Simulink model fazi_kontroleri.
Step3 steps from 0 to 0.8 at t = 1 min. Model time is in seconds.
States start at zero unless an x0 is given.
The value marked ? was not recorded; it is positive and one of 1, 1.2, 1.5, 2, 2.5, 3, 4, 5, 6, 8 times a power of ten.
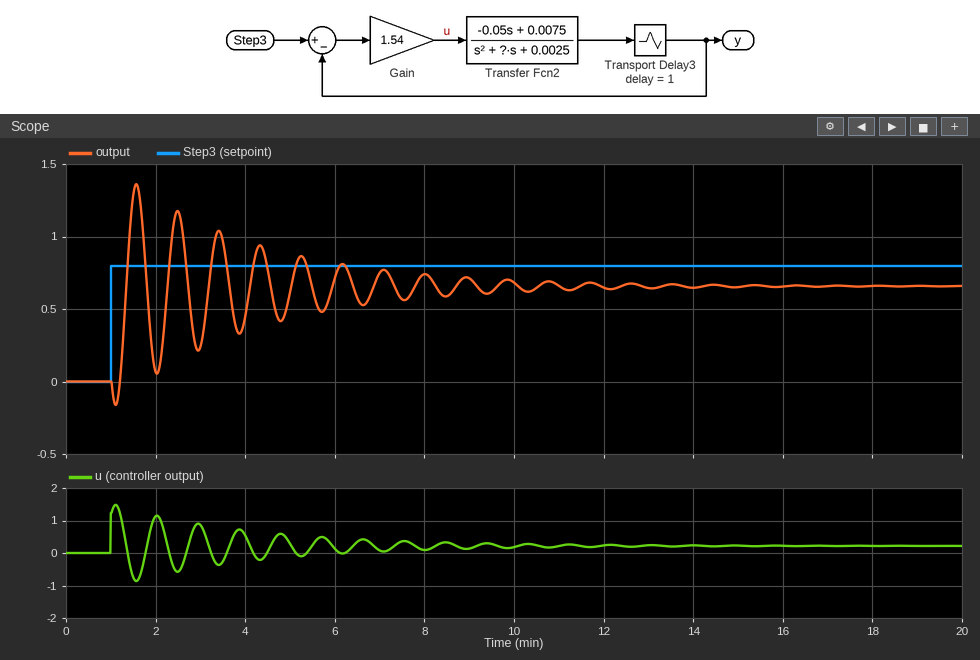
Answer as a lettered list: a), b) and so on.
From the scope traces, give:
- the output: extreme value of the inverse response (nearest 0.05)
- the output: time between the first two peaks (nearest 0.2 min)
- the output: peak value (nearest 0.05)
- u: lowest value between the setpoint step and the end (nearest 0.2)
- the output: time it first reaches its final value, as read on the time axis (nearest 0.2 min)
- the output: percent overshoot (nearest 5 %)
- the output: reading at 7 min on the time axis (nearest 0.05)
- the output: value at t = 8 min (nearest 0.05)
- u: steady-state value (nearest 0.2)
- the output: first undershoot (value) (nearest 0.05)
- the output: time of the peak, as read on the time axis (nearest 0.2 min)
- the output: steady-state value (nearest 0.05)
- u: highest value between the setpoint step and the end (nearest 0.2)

a) -0.15
b) 1.0 min
c) 1.35
d) -0.8
e) 1.4 min
f) 105 %
g) 0.75
h) 0.75
i) 0.2
j) 0.05
k) 1.6 min
l) 0.65
m) 1.4
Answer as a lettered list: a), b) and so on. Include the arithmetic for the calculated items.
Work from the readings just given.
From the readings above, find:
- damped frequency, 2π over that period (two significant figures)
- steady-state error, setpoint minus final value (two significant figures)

a) 2π / 1 = 6.3 rad/min
b) 0.8 - 0.65 = 0.15
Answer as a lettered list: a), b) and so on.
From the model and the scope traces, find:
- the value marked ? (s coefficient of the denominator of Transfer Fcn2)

a) 0.1
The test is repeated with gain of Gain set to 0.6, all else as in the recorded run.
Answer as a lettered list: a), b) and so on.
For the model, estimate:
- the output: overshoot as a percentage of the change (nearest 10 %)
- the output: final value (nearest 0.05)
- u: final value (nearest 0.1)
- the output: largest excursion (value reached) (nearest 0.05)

a) 30 %
b) 0.50
c) 0.2
d) 0.65
